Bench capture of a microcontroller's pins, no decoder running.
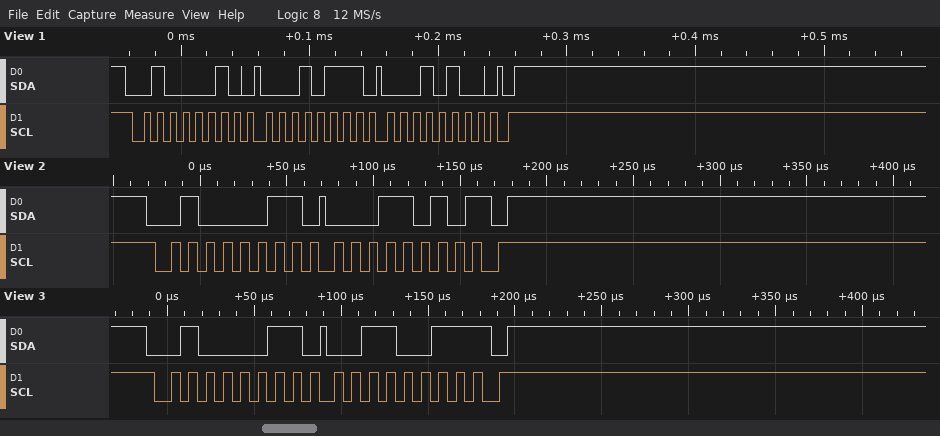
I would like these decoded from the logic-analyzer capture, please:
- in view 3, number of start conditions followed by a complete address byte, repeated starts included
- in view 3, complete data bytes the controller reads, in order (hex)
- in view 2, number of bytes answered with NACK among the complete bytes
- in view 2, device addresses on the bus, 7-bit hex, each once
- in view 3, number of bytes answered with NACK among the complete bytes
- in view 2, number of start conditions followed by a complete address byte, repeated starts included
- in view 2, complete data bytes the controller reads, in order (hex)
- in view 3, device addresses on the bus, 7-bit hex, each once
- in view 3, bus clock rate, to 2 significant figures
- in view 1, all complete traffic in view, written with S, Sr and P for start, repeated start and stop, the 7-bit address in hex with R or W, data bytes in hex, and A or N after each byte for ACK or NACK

1
33
1
0x21
1
1
1A
0x21
100 kHz
S 21W A 17 A 14 A P
